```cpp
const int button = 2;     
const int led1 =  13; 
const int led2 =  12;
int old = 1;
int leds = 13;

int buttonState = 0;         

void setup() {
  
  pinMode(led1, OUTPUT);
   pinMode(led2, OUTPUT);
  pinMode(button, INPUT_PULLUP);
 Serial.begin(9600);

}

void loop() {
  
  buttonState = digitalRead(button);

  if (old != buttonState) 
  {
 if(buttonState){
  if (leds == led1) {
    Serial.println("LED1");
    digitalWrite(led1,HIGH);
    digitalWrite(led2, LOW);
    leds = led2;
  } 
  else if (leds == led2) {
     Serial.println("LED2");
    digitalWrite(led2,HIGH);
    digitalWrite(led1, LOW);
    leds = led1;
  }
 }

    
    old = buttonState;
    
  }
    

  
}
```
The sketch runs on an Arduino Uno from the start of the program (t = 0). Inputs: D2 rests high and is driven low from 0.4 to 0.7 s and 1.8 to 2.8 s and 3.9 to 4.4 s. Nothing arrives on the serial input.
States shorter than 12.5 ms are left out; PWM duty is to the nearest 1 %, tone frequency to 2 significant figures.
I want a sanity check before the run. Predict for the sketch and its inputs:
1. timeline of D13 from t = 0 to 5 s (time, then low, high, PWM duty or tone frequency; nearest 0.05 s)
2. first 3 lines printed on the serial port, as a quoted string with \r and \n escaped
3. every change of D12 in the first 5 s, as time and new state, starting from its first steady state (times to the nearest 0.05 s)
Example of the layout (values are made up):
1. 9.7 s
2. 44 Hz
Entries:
1. 0 s low; 0.7 s high; 2.8 s low; 4.4 s high
2. "LED1\r\nLED2\r\nLED1\r\n"
3. 0 s low; 2.8 s high; 4.4 s low
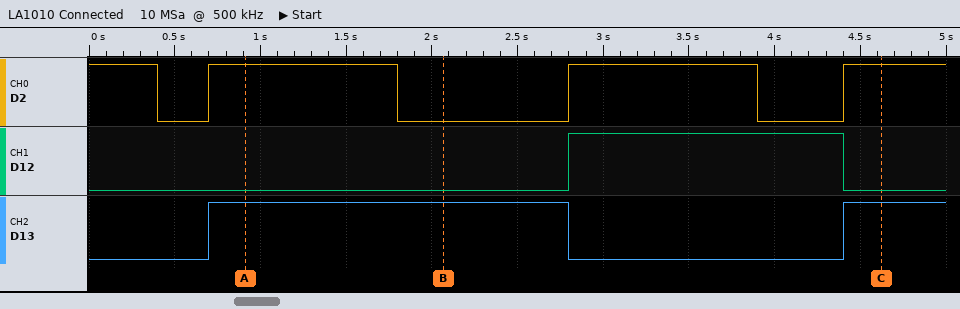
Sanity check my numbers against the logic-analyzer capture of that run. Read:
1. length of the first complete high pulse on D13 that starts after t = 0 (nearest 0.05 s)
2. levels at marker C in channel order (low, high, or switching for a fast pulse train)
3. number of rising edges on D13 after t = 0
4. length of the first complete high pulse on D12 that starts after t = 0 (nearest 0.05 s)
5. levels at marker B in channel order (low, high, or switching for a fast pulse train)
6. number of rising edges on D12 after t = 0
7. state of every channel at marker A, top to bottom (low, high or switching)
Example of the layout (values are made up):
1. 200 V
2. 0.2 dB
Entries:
1. 2.10 s
2. D2 high, D12 low, D13 high
3. 2
4. 1.60 s
5. D2 low, D12 low, D13 high
6. 1
7. D2 high, D12 low, D13 high
